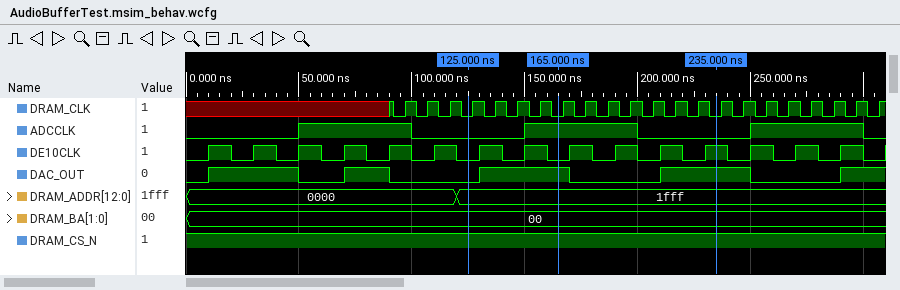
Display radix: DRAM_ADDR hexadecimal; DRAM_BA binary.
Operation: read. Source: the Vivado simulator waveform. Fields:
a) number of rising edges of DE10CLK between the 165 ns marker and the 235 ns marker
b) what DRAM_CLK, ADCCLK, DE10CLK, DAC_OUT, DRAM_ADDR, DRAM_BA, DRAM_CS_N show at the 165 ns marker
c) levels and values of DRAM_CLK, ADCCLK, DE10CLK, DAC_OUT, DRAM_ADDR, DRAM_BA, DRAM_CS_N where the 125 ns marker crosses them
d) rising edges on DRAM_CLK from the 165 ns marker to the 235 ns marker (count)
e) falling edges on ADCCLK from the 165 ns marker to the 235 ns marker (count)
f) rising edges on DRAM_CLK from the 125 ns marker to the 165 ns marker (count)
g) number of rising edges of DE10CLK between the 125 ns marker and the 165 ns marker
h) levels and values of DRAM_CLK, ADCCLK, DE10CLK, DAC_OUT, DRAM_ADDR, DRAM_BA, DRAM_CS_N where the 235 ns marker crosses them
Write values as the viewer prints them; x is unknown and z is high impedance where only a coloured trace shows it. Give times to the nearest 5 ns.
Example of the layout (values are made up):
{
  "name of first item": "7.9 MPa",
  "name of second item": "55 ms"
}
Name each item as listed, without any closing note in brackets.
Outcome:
{
  "number of rising edges of DE10CLK between the 165 ns marker and the 235 ns marker": "4",
  "what DRAM_CLK, ADCCLK, DE10CLK, DAC_OUT, DRAM_ADDR, DRAM_BA, DRAM_CS_N show at the 165 ns marker": "DRAM_CLK=0, ADCCLK=1, DE10CLK=0, DAC_OUT=1, DRAM_ADDR=1fff, DRAM_BA=00, DRAM_CS_N=1",
  "levels and values of DRAM_CLK, ADCCLK, DE10CLK, DAC_OUT, DRAM_ADDR, DRAM_BA, DRAM_CS_N where the 125 ns marker crosses them": "DRAM_CLK=0, ADCCLK=0, DE10CLK=0, DAC_OUT=0, DRAM_ADDR=1fff, DRAM_BA=00, DRAM_CS_N=1",
  "rising edges on DRAM_CLK from the 165 ns marker to the 235 ns marker": "7",
  "falling edges on ADCCLK from the 165 ns marker to the 235 ns marker": "1",
  "rising edges on DRAM_CLK from the 125 ns marker to the 165 ns marker": "4",
  "number of rising edges of DE10CLK between the 125 ns marker and the 165 ns marker": "2",
  "levels and values of DRAM_CLK, ADCCLK, DE10CLK, DAC_OUT, DRAM_ADDR, DRAM_BA, DRAM_CS_N where the 235 ns marker crosses them": "DRAM_CLK=0, ADCCLK=0, DE10CLK=1, DAC_OUT=1, DRAM_ADDR=1fff, DRAM_BA=00, DRAM_CS_N=1"
}
